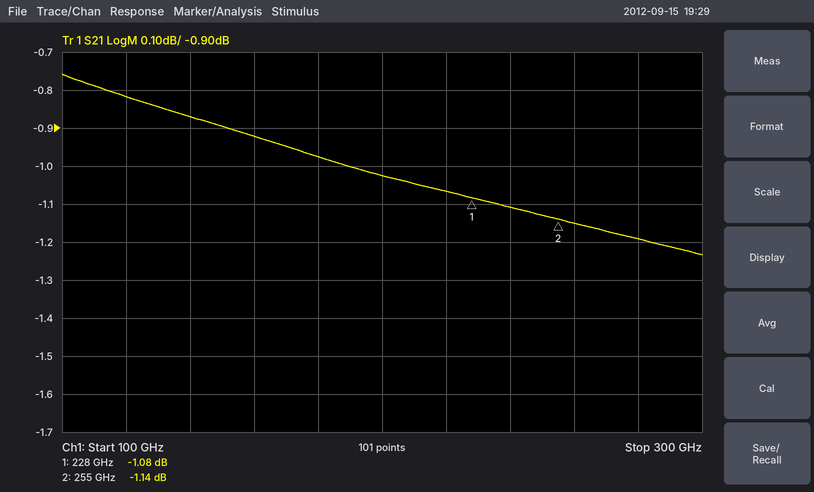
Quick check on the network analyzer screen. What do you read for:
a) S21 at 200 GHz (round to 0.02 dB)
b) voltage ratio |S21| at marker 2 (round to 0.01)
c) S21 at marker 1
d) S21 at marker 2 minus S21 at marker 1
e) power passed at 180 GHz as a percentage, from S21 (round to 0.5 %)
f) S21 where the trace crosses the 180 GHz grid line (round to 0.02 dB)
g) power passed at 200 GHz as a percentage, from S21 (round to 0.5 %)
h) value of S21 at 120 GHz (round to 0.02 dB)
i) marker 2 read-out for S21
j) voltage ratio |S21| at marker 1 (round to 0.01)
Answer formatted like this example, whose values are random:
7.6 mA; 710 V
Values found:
-1.02 dB; 0.88; -1.08 dB; -0.06 dB; 80.0 %; -0.98 dB; 79.0 %; -0.82 dB; -1.14 dB; 0.88
